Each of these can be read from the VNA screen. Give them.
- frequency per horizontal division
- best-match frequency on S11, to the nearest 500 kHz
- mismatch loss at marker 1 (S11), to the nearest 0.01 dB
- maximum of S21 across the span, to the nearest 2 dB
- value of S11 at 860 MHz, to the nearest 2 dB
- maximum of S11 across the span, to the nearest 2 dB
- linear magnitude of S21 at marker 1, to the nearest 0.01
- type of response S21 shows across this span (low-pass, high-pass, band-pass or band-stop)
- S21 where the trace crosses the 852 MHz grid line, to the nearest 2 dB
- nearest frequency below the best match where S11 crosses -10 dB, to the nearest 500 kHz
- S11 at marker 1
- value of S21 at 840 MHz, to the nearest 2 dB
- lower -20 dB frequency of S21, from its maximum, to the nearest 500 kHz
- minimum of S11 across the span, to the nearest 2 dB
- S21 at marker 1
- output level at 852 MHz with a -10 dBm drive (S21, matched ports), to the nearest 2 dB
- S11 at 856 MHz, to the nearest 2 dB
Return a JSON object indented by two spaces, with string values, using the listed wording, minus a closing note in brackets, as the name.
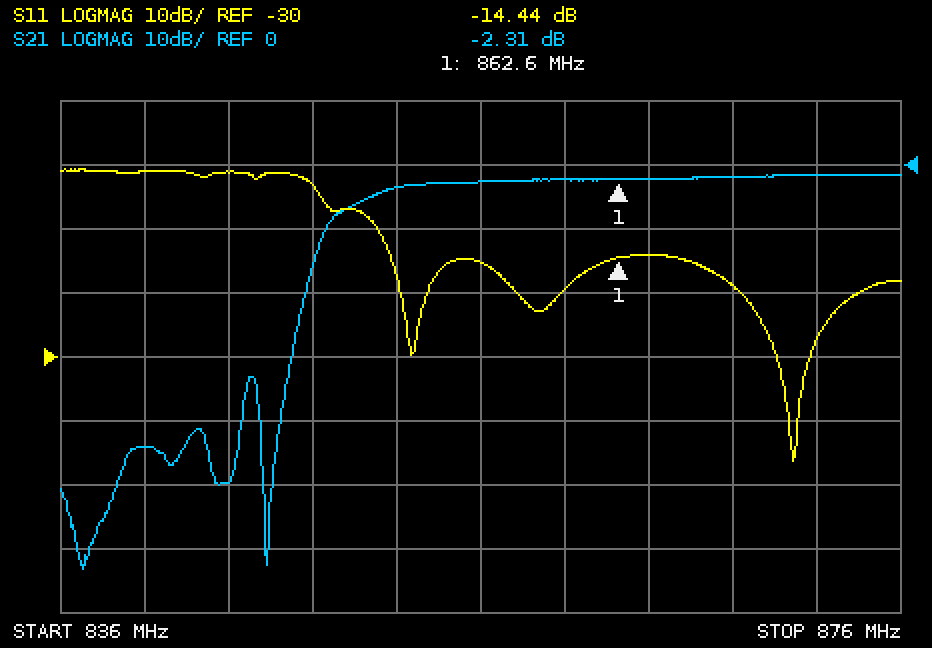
{
  "frequency per horizontal division": "4 MHz",
  "best-match frequency on S11, to the nearest 500 kHz": "871.0 MHz",
  "mismatch loss at marker 1 (S11), to the nearest 0.01 dB": "0.16 dB",
  "maximum of S21 across the span, to the nearest 2 dB": "-2 dB",
  "value of S11 at 860 MHz, to the nearest 2 dB": "-20 dB",
  "maximum of S11 across the span, to the nearest 2 dB": "0 dB",
  "linear magnitude of S21 at marker 1, to the nearest 0.01": "0.77",
  "type of response S21 shows across this span": "high-pass",
  "S21 where the trace crosses the 852 MHz grid line, to the nearest 2 dB": "-4 dB",
  "nearest frequency below the best match where S11 crosses -10 dB, to the nearest 500 kHz": "851.0 MHz",
  "S11 at marker 1": "-14.44 dB",
  "value of S21 at 840 MHz, to the nearest 2 dB": "-44 dB",
  "lower -20 dB frequency of S21, from its maximum, to the nearest 500 kHz": "847.5 MHz",
  "minimum of S11 across the span, to the nearest 2 dB": "-46 dB",
  "S21 at marker 1": "-2.31 dB",
  "output level at 852 MHz with a -10 dBm drive (S21, matched ports), to the nearest 2 dB": "-14 dBm",
  "S11 at 856 MHz, to the nearest 2 dB": "-16 dB"
}
